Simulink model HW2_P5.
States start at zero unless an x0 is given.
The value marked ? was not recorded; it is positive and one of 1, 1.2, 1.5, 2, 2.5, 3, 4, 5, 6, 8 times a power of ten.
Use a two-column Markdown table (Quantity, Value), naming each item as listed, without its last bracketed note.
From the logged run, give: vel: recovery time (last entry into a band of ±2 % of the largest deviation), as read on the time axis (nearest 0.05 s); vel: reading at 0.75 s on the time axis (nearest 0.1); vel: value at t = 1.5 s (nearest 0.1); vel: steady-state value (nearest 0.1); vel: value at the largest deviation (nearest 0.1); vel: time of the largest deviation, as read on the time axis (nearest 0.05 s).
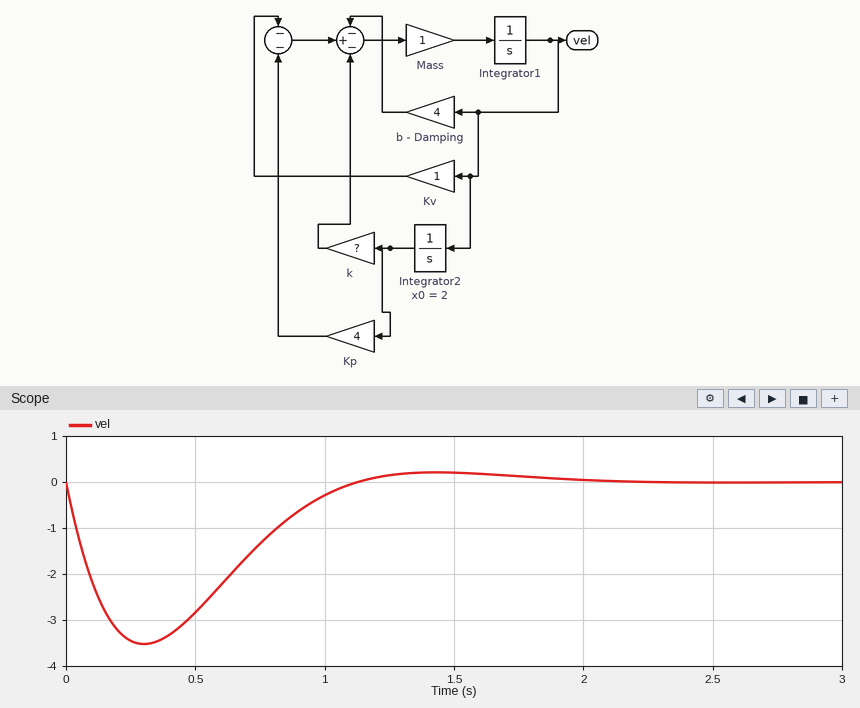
| Quantity | Value |
|---|---|
| vel: recovery time (last entry into a band of ±2 % of the largest deviation), as read on the time axis | 1.90 s |
| vel: reading at 0.75 s on the time axis | -1.3 |
| vel: value at t = 1.5 s | 0.2 |
| vel: steady-state value | 0.0 |
| vel: value at the largest deviation | -3.5 |
| vel: time of the largest deviation, as read on the time axis | 0.30 s |
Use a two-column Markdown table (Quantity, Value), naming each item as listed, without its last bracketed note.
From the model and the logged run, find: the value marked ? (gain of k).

| Quantity | Value |
|---|---|
| the value marked ? | 10 |
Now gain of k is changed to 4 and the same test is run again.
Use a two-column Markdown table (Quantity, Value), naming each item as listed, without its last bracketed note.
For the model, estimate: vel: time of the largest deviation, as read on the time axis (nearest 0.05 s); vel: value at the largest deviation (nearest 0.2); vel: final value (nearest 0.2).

| Quantity | Value |
|---|---|
| vel: time of the largest deviation, as read on the time axis | 0.35 s |
| vel: value at the largest deviation | -2.2 |
| vel: final value | 0.0 |
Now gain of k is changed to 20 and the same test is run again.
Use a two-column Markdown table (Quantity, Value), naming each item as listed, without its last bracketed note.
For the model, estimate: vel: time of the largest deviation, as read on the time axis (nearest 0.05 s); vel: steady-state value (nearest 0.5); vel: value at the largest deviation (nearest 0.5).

| Quantity | Value |
|---|---|
| vel: time of the largest deviation, as read on the time axis | 0.25 s |
| vel: steady-state value | 0.0 |
| vel: value at the largest deviation | -5.5 |
